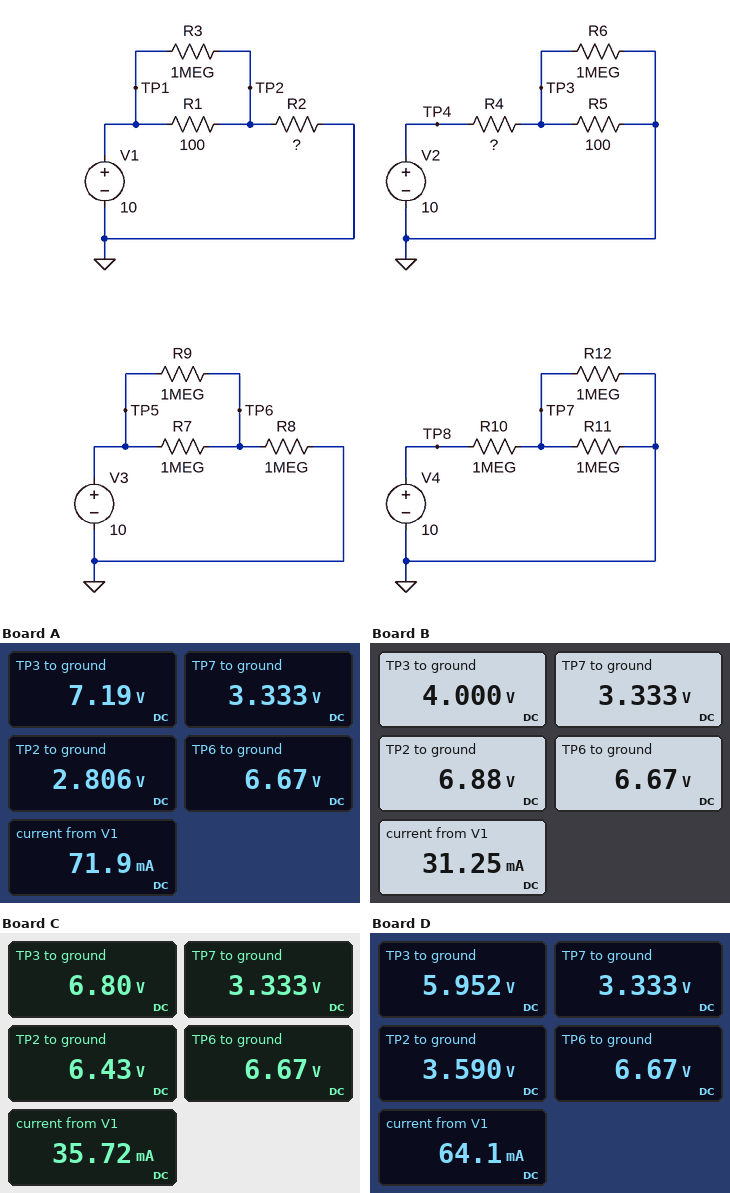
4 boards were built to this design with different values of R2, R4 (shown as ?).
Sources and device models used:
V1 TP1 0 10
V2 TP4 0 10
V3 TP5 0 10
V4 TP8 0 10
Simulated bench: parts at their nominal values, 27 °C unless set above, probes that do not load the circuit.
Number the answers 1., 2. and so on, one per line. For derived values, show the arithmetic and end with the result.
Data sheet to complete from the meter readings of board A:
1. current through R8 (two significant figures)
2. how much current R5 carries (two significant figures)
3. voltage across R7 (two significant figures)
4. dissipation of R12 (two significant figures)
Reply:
1. (6.67 V) / 1 MΩ = 6.7 µA
2. (7.19 V) / 100 Ω = 72 mA
3. 10 V - 6.67 V = 3.3 V
4. (3.333 V)^2 / 1 MΩ = 11 µW
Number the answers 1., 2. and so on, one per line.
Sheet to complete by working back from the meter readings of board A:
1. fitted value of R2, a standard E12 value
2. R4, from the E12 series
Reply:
1. 39 Ω
2. 39 Ω
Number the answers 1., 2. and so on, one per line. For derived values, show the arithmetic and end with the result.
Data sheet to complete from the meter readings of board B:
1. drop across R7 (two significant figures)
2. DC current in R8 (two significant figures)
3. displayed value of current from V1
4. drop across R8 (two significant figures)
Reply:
1. 10 V - 6.67 V = 3.3 V
2. (6.67 V) / 1 MΩ = 6.7 µA
3. 31.25 mA
4. 6.67 V = 6.7 V
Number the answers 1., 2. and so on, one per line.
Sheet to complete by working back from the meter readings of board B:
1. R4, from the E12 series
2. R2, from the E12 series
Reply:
1. 150 Ω
2. 220 Ω
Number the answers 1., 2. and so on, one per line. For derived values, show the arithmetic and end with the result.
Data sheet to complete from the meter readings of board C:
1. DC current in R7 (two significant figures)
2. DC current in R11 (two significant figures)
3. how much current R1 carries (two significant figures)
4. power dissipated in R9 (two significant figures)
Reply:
1. (10 V - 6.67 V) / 1 MΩ = 3.3 µA
2. (3.333 V) / 1 MΩ = 3.3 µA
3. (10 V - 6.43 V) / 100 Ω = 36 mA
4. (10 V - 6.67 V)^2 / 1 MΩ = 11 µW
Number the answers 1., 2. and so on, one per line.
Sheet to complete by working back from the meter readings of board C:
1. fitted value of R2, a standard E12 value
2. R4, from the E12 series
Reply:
1. 180 Ω
2. 47 Ω
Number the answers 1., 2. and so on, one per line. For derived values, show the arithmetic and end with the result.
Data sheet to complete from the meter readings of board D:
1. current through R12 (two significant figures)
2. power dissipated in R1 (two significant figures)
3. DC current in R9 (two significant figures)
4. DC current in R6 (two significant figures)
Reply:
1. (3.333 V) / 1 MΩ = 3.3 µA
2. (10 V - 3.59 V)^2 / 100 Ω = 410 mW
3. (10 V - 6.67 V) / 1 MΩ = 3.3 µA
4. (5.952 V) / 1 MΩ = 6.0 µA
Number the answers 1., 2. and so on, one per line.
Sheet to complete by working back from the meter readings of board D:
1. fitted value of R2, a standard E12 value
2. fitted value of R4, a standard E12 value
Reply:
1. 56 Ω
2. 68 Ω
